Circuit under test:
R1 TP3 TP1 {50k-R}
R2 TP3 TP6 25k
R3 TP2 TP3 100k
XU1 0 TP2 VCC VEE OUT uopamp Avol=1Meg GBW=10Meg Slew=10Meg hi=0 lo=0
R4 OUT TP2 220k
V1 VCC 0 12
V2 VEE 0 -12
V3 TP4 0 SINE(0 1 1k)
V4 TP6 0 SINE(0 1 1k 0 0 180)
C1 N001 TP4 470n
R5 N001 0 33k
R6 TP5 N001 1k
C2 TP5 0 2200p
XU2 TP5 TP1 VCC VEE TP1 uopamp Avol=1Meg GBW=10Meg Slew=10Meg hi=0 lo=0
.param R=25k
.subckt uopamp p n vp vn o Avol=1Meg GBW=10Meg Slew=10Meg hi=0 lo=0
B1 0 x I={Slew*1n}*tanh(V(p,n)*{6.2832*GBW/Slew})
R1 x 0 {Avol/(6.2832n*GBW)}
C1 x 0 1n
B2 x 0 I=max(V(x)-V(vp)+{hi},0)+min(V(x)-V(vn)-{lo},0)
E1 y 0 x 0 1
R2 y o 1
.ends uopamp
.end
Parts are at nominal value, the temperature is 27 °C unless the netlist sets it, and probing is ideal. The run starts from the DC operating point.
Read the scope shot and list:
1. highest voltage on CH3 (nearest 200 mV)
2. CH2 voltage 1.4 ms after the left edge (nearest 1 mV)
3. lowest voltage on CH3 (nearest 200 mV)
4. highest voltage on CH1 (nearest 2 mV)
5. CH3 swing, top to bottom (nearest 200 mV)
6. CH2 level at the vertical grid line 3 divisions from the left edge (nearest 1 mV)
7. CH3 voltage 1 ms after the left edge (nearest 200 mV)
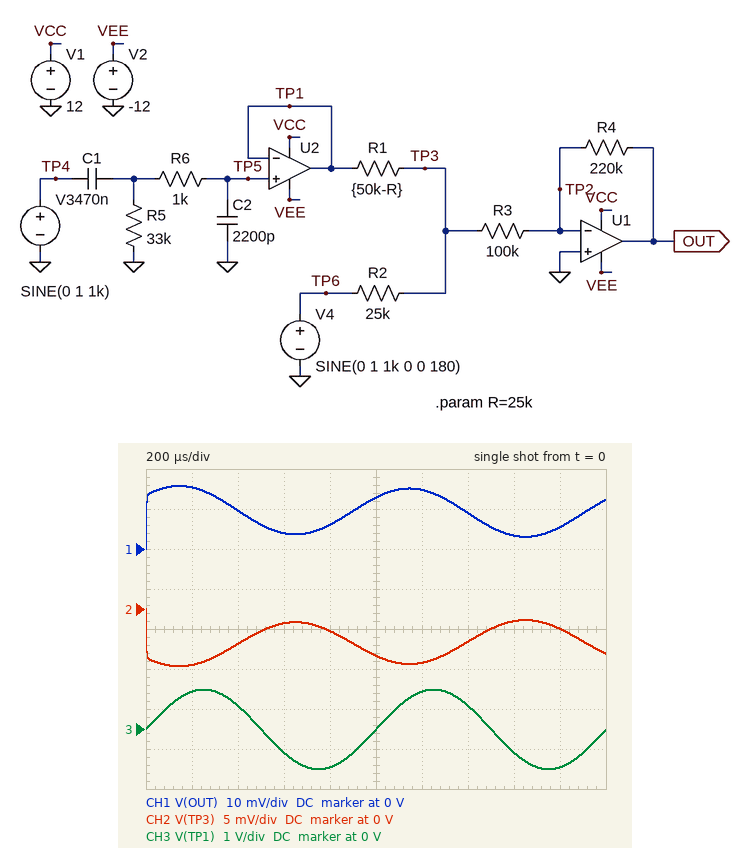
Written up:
1.0 V
-4 mV
-1.0 V
16 mV
2.0 V
-2 mV
0 V
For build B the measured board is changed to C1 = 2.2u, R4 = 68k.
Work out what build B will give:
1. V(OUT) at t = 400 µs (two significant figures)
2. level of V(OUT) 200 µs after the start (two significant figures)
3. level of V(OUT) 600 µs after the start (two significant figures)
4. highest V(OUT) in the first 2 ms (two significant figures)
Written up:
-2.0 mV
2.1 mV
-2.4 mV
4.2 mV
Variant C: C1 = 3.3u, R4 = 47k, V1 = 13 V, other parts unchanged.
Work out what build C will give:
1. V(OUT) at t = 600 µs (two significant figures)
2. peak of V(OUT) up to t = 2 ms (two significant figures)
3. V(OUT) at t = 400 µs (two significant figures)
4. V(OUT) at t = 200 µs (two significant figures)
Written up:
-1.9 mV
2.9 mV
-1.7 mV
1.3 mV
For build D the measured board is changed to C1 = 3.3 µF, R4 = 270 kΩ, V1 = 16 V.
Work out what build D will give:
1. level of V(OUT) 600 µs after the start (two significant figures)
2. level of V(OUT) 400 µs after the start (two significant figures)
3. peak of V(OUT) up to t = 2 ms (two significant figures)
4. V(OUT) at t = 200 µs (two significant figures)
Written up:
-11 mV
-9.7 mV
17 mV
7.3 mV
